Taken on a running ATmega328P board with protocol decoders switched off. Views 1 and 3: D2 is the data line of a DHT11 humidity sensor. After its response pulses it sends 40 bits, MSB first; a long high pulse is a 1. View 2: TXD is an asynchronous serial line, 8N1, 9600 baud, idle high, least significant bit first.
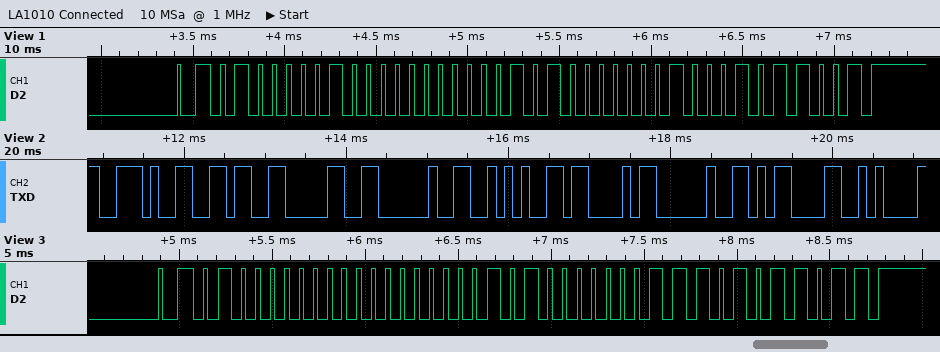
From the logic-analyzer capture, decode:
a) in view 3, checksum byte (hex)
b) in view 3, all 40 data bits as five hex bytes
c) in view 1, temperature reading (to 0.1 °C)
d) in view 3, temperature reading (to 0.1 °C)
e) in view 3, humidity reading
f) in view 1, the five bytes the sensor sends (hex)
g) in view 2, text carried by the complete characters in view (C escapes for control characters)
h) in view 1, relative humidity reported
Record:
0x5B
40 00 14 07 5B
20.4 °C
20.7 °C
64 %
41 00 14 04 59
".60 *C \r\n"
65 %
